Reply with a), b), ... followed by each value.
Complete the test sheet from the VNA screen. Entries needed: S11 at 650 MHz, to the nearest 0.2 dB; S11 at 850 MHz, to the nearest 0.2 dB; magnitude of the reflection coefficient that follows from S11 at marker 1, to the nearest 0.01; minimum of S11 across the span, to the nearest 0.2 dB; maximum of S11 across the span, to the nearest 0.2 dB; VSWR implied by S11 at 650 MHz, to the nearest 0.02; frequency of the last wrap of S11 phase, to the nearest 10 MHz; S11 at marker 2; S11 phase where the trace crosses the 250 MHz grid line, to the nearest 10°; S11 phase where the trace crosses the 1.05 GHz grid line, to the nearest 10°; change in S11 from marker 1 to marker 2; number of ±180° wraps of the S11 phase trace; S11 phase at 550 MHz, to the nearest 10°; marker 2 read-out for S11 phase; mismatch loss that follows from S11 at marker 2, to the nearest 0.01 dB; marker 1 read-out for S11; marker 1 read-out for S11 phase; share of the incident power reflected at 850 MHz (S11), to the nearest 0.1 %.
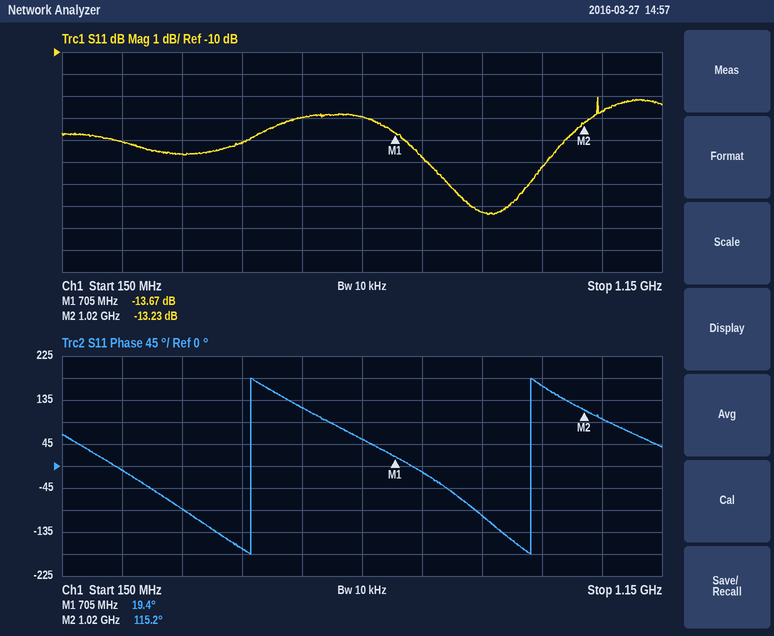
a) -13.0 dB
b) -17.2 dB
c) 0.21
d) -17.4 dB
e) -12.0 dB
f) 1.58
g) 930 MHz
h) -13.23 dB
i) -10°
j) 100°
k) 0.44 dB
l) 2
m) 120°
n) 115.2°
o) 0.21 dB
p) -13.67 dB
q) 19.4°
r) 1.9 %
